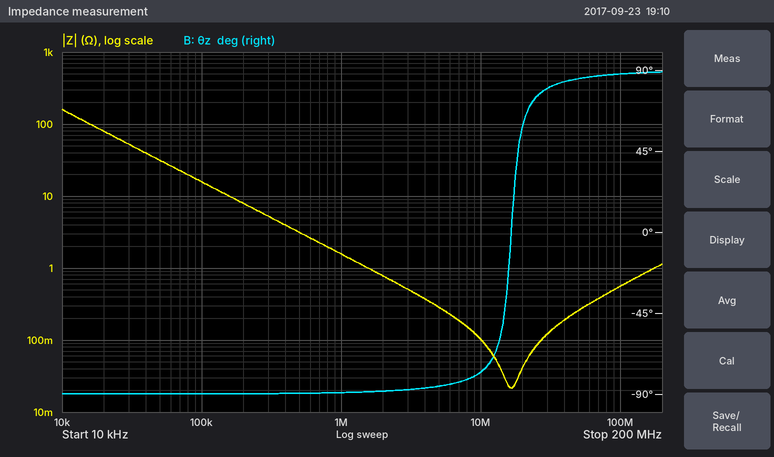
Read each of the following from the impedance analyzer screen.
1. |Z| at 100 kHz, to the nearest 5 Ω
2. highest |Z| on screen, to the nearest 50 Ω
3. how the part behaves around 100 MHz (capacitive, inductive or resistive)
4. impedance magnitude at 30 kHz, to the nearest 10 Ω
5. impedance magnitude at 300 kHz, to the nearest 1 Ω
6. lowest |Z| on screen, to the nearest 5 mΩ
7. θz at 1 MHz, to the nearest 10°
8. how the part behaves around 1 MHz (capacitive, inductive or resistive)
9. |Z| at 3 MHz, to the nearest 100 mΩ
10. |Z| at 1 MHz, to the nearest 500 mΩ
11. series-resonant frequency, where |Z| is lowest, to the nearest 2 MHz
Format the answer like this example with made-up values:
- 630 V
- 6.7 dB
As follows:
- 15 Ω
- 150 Ω
- inductive
- 50 Ω
- 5 Ω
- 20 mΩ
- -90°
- capacitive
- 500 mΩ
- 1.5 Ω
- 16 MHz
